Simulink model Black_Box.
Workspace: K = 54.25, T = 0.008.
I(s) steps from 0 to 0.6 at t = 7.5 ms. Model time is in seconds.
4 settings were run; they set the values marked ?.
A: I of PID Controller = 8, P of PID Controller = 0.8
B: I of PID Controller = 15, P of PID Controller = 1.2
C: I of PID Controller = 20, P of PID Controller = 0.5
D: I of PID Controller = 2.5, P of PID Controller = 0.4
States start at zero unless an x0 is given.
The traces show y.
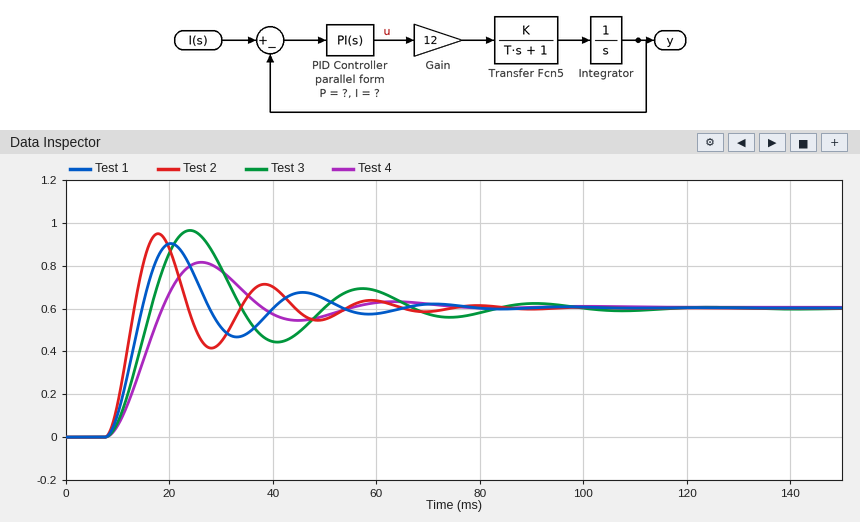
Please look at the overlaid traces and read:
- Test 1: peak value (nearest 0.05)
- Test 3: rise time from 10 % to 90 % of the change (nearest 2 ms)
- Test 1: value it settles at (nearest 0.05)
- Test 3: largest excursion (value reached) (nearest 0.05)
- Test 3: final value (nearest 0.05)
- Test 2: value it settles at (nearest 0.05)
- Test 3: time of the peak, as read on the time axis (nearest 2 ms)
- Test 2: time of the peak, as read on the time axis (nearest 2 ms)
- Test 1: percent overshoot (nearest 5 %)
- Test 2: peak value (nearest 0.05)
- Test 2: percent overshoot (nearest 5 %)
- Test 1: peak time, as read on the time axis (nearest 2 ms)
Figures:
0.90
6 ms
0.60
0.95
0.60
0.60
24 ms
18 ms
50 %
0.95
60 %
20 ms
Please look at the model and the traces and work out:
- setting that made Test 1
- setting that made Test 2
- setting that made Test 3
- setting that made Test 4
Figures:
A
B
C
D
